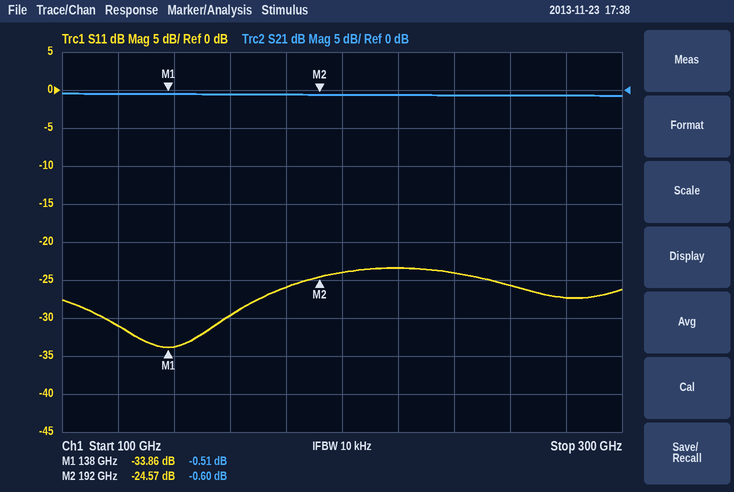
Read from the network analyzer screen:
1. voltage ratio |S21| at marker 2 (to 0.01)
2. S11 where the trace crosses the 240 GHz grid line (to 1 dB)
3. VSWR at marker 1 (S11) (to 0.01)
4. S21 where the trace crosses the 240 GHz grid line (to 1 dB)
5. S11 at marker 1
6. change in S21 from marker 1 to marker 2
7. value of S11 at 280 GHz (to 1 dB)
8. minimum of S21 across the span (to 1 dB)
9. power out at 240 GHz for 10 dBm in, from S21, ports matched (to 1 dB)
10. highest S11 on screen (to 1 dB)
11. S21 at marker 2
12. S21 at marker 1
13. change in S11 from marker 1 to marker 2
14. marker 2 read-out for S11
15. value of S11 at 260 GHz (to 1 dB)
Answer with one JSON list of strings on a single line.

["0.93", "-24 dB", "1.04", "-1 dB", "-33.86 dB", "-0.09 dB", "-27 dB", "-1 dB", "9 dBm", "-23 dB", "-0.60 dB", "-0.51 dB", "9.29 dB", "-24.57 dB", "-26 dB"]
